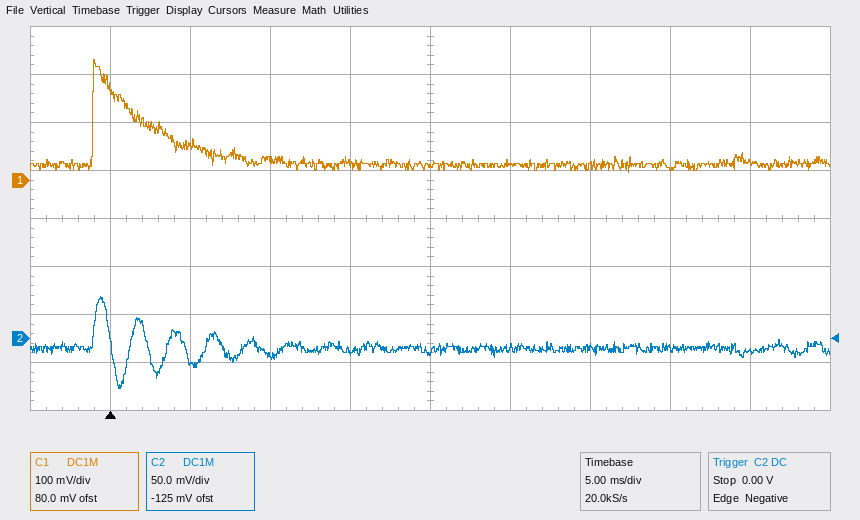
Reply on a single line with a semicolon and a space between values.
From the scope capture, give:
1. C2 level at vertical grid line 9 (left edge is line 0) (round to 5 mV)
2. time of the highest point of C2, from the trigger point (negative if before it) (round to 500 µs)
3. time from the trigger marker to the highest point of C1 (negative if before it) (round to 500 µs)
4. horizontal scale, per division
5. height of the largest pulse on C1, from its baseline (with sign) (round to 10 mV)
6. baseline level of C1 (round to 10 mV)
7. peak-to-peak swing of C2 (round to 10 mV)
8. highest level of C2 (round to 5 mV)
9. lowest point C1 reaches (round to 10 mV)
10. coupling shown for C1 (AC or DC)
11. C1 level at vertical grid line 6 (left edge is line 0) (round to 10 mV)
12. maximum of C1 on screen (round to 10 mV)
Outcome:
-15 mV; -500 µs; -1.0 ms; 5 ms; +220 mV; 30 mV; 100 mV; 45 mV; 20 mV; DC; 40 mV; 250 mV
